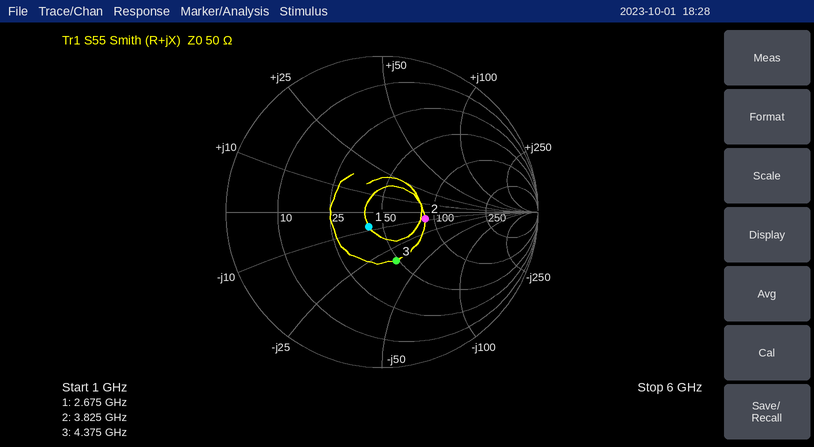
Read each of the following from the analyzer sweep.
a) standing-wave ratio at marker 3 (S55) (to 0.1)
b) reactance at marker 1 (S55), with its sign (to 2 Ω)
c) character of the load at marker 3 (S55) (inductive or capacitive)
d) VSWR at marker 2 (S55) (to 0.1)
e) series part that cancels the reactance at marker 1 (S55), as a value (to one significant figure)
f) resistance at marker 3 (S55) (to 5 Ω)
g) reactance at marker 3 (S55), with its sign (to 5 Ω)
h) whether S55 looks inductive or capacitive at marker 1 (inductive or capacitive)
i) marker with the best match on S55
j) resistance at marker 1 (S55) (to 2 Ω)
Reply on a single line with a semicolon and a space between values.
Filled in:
2.0; -8 Ω; capacitive; 1.8; 500 pH; 50 Ω; -35 Ω; capacitive; marker 1; 42 Ω
